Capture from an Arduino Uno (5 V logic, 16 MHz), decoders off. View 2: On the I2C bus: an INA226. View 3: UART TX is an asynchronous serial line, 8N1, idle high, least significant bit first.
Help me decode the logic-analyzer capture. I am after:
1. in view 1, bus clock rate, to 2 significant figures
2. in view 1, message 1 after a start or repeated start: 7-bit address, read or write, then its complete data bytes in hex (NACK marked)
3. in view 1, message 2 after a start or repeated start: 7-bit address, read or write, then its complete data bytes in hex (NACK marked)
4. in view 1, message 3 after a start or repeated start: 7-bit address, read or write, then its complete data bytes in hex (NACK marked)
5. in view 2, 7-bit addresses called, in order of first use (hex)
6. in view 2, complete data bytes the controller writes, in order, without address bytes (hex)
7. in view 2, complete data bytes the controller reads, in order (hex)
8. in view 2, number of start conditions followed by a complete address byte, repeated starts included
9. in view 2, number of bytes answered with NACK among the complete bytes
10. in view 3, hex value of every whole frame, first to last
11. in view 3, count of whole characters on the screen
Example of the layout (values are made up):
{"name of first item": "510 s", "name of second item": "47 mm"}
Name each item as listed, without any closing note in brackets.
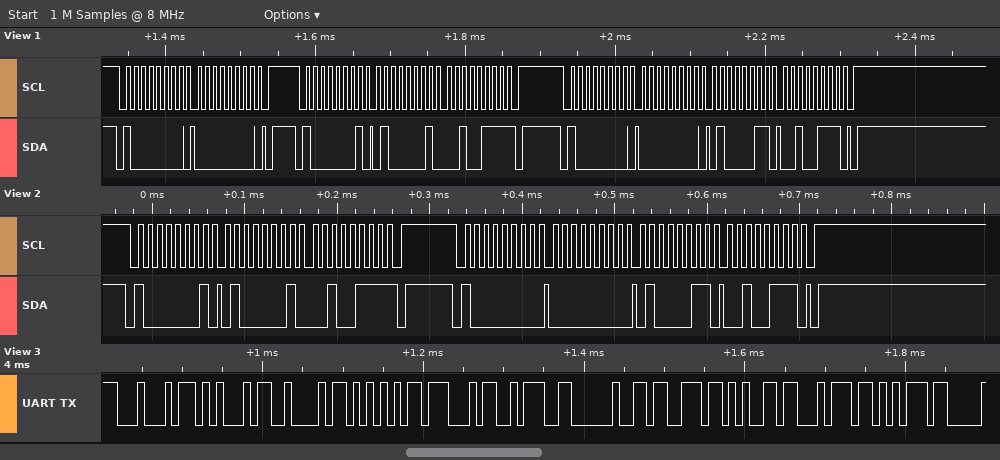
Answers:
{"in view 1, bus clock rate, to 2 significant figures": "100 kHz", "in view 1, message 1 after a start or repeated start: 7-bit address, read or write, then its complete data bytes in hex": "0x40 write: 00", "in view 1, message 2 after a start or repeated start: 7-bit address, read or write, then its complete data bytes in hex": "0x40 read: 41 27 NACK", "in view 1, message 3 after a start or repeated start: 7-bit address, read or write, then its complete data bytes in hex": "0x40 write: 00 43 27", "in view 2, 7-bit addresses called, in order of first use": "0x40", "in view 2, complete data bytes the controller writes, in order, without address bytes": "00 43 27", "in view 2, complete data bytes the controller reads, in order": "41 27", "in view 2, number of start conditions followed by a complete address byte, repeated starts included": "2", "in view 2, number of bytes answered with NACK among the complete bytes": "1", "in view 3, hex value of every whole frame, first to last": "44 45 42 55 47 3A 20 73 65 74 75", "in view 3, count of whole characters on the screen": "11"}
